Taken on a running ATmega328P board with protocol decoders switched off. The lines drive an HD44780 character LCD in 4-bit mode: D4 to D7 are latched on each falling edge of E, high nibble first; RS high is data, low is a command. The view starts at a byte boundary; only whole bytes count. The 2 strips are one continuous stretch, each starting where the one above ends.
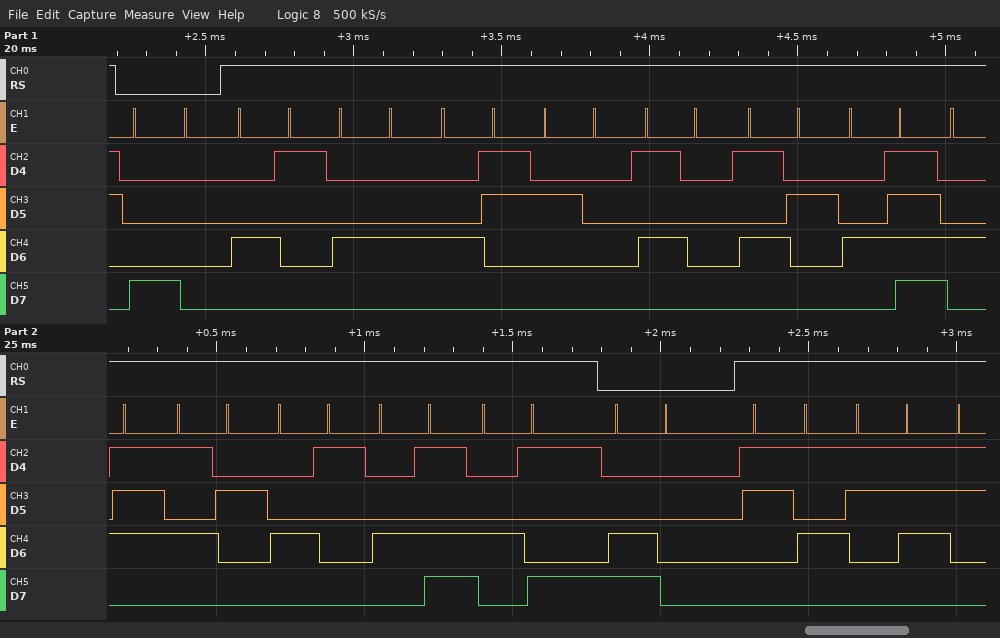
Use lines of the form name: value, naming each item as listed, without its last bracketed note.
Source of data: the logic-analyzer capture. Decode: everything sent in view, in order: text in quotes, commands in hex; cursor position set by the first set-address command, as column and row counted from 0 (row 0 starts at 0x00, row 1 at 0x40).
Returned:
everything sent in view, in order: text in quotes, commands in hex: 0x80 "ADC PROGRAMI" 0xC0 "57"
cursor position set by the first set-address command, as column and row counted from 0: column 0, row 0
